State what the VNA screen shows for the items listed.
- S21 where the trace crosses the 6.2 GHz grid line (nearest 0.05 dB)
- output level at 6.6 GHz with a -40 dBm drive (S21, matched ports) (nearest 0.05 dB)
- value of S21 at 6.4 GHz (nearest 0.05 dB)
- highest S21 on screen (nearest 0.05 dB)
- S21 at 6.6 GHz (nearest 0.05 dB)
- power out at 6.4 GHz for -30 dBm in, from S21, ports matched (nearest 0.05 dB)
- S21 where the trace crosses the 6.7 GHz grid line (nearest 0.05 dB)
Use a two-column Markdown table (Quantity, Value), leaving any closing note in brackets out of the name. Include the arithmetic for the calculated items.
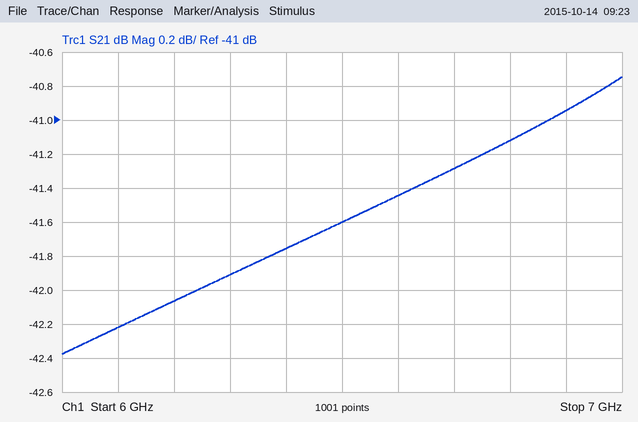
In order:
| Quantity | Value |
|---|---|
| S21 where the trace crosses the 6.2 GHz grid line | -42.05 dB |
| output level at 6.6 GHz with a -40 dBm drive (S21, matched ports) | -40 dBm + (-41.45 dB) = -81.45 dBm |
| value of S21 at 6.4 GHz | -41.75 dB |
| highest S21 on screen | -40.75 dB |
| S21 at 6.6 GHz | -41.45 dB |
| power out at 6.4 GHz for -30 dBm in, from S21, ports matched | -30 dBm + (-41.75 dB) = -71.75 dBm |
| S21 where the trace crosses the 6.7 GHz grid line | -41.30 dB |
